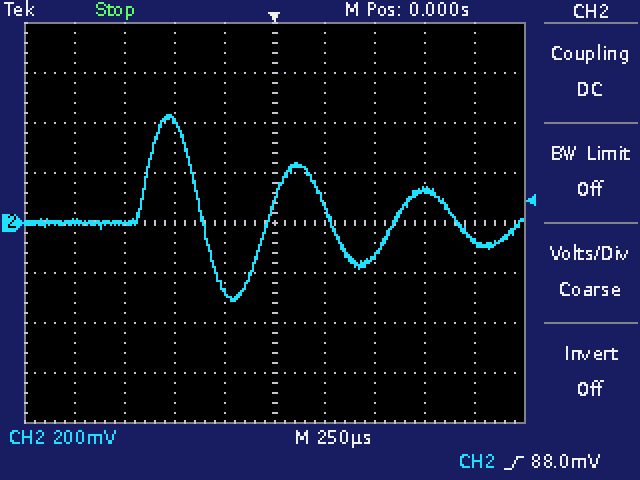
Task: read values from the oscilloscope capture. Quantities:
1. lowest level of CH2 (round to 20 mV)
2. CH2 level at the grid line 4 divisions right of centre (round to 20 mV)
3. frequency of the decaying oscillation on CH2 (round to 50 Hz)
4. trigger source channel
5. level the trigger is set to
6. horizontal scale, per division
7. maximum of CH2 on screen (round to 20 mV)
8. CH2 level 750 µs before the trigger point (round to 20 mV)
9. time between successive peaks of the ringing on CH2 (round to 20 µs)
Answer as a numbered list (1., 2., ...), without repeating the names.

1. -320 mV
2. -80 mV
3. 1.55 kHz
4. CH2
5. 88.0 mV
6. 250 µs
7. 440 mV
8. 0 mV
9. 640 µs
